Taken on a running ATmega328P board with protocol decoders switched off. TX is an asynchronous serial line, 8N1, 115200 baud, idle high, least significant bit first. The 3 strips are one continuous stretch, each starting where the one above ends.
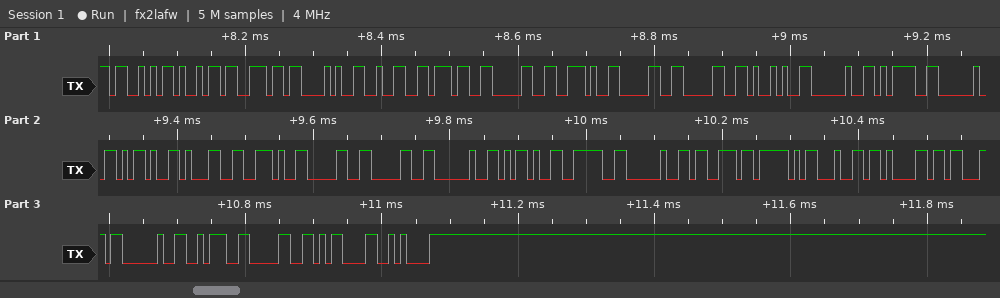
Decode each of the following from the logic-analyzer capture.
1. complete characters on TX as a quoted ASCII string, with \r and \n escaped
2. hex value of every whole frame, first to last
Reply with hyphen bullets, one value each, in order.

- "Sin(270.00) = -1.00 -> s_dac :0\r\n"
- 53 69 6E 28 32 37 30 2E 30 30 29 20 3D 20 2D 31 2E 30 30 20 2D 3E 20 73 5F 64 61 63 20 3A 30 0D 0A
